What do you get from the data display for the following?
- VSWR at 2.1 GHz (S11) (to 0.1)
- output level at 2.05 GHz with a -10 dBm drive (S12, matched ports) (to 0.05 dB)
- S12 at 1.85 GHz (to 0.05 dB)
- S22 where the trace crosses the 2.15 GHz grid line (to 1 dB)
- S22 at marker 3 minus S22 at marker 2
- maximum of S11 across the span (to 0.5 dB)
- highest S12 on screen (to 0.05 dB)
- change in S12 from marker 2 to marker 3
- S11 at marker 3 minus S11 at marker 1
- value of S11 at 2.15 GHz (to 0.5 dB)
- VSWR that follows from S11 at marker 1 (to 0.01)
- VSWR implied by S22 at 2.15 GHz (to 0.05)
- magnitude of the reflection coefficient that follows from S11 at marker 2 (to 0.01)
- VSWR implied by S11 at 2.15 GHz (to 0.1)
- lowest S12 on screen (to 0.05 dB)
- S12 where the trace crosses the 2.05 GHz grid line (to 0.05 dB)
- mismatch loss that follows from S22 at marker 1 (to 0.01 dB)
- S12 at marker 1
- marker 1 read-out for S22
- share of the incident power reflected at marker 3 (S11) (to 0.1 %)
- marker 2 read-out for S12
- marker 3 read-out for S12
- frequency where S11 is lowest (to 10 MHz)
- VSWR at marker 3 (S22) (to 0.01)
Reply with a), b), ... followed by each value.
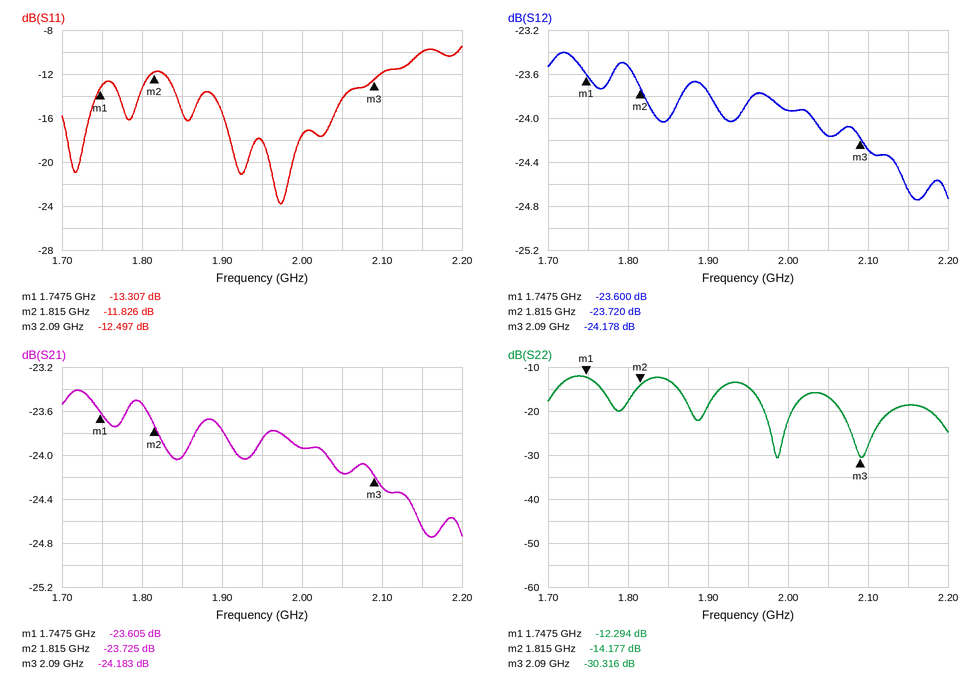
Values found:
a) 1.7
b) -34.15 dBm
c) -24.00 dB
d) -19 dB
e) -16.139 dB
f) -9.5 dB
g) -23.40 dB
h) -0.458 dB
i) 0.810 dB
j) -10.0 dB
k) 1.55
l) 1.25
m) 0.26
n) 1.9
o) -24.75 dB
p) -24.15 dB
q) 0.26 dB
r) -23.600 dB
s) -12.294 dB
t) 5.6 %
u) -23.720 dB
v) -24.178 dB
w) 1.97 GHz
x) 1.06
